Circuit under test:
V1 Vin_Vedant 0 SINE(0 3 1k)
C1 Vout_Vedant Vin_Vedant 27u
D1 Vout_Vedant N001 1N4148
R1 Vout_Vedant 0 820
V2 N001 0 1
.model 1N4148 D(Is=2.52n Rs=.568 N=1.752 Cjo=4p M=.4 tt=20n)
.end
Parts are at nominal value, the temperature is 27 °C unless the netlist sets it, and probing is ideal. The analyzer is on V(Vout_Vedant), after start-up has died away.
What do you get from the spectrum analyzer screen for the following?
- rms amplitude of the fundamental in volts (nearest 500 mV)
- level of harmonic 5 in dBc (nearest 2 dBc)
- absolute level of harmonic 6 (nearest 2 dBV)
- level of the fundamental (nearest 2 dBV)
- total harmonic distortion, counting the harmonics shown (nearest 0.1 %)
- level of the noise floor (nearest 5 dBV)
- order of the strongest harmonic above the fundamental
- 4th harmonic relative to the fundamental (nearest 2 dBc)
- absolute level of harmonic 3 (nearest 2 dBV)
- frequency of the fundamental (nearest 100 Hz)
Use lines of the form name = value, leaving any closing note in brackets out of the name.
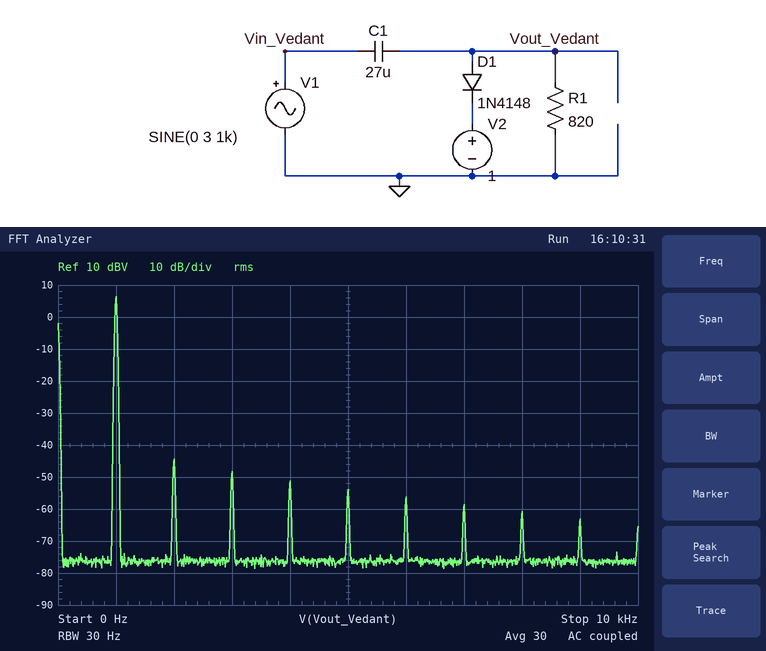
rms amplitude of the fundamental in volts = 2.0 V
level of harmonic 5 in dBc = -60 dBc
absolute level of harmonic 6 = -56 dBV
level of the fundamental = 6 dBV
total harmonic distortion, counting the harmonics shown = 0.4 %
level of the noise floor = -75 dBV
order of the strongest harmonic above the fundamental = 2
4th harmonic relative to the fundamental = -58 dBc
absolute level of harmonic 3 = -48 dBV
frequency of the fundamental = 1.0 kHz
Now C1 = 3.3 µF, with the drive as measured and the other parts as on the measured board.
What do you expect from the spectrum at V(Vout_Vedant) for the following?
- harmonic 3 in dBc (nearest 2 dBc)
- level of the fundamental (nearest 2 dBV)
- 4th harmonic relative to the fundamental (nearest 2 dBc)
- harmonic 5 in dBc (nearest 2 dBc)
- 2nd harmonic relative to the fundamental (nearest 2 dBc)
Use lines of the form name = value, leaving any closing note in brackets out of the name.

harmonic 3 in dBc = -38 dBc
level of the fundamental = 6 dBV
4th harmonic relative to the fundamental = -40 dBc
harmonic 5 in dBc = -44 dBc
2nd harmonic relative to the fundamental = -34 dBc
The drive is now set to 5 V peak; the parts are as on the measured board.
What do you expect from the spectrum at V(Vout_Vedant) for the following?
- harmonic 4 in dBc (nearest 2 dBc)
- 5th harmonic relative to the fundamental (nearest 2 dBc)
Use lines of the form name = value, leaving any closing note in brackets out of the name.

harmonic 4 in dBc = -54 dBc
5th harmonic relative to the fundamental = -56 dBc
